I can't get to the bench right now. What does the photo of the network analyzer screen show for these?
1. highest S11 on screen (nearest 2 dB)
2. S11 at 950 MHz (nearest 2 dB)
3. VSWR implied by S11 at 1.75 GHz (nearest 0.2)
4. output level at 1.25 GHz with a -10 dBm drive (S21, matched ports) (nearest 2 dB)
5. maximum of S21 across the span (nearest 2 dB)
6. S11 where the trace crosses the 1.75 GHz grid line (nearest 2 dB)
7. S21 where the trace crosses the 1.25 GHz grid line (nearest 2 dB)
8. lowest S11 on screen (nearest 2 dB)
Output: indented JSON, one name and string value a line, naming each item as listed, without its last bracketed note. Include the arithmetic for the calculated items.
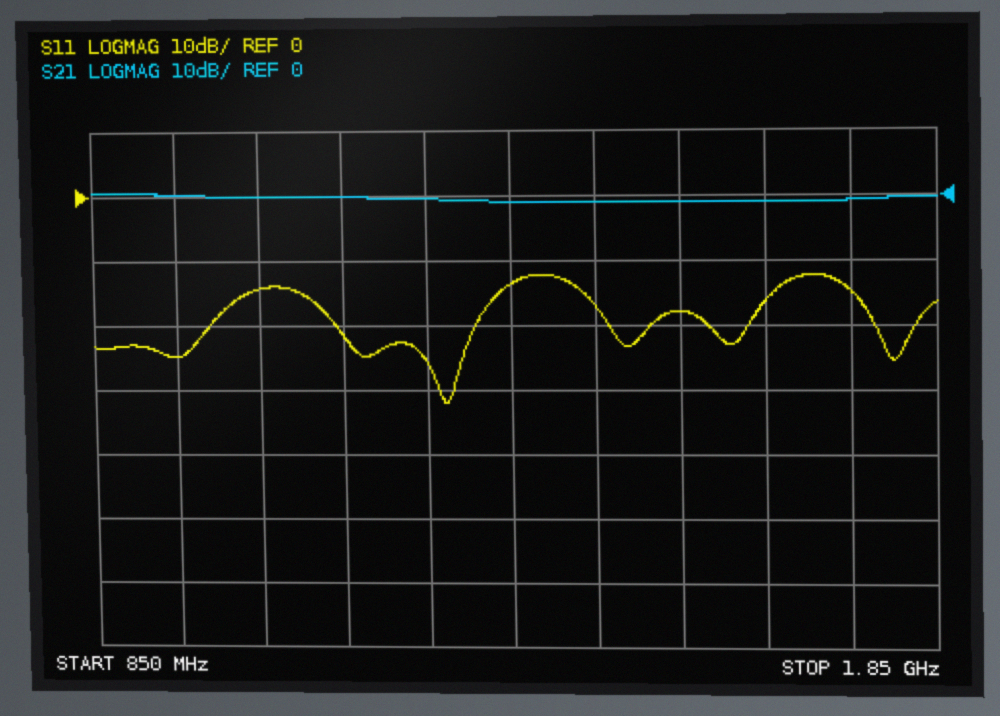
{
  "highest S11 on screen": "-12 dB",
  "S11 at 950 MHz": "-24 dB",
  "VSWR implied by S11 at 1.75 GHz": "|Γ| = 10^(-14/20) = 0.1995; VSWR = (1 + 0.1995)/(1 − 0.1995) ≈ 1.50, so 1.4 to the nearest 0.2",
  "output level at 1.25 GHz with a -10 dBm drive (S21, matched ports)": "-10 dBm + (0 dB) = -10 dBm",
  "maximum of S21 across the span": "0 dB",
  "S11 where the trace crosses the 1.75 GHz grid line": "-14 dB",
  "S21 where the trace crosses the 1.25 GHz grid line": "0 dB",
  "lowest S11 on screen": "-32 dB"
}
